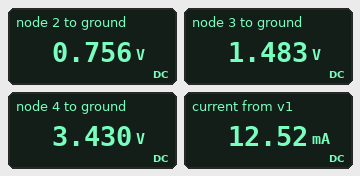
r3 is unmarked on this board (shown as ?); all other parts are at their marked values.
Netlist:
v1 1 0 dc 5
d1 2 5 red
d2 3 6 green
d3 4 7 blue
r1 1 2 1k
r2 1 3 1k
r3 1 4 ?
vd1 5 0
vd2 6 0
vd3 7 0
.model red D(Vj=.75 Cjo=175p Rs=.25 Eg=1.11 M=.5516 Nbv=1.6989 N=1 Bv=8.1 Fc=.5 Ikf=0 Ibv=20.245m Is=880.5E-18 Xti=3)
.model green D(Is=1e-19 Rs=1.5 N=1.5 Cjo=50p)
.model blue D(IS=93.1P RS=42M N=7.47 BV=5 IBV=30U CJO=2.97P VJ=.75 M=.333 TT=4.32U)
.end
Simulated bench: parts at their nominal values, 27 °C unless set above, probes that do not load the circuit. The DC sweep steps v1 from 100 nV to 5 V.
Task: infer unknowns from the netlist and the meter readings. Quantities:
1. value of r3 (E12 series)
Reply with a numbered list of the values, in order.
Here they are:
1. 330 Ω
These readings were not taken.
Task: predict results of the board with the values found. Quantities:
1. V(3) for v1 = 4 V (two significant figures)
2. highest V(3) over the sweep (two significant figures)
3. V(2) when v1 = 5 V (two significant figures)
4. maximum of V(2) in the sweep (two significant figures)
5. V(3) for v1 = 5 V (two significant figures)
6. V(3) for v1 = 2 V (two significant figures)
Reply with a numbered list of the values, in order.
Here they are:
1. 1.5 V
2. 1.5 V
3. 760 mV
4. 760 mV
5. 1.5 V
6. 1.4 V
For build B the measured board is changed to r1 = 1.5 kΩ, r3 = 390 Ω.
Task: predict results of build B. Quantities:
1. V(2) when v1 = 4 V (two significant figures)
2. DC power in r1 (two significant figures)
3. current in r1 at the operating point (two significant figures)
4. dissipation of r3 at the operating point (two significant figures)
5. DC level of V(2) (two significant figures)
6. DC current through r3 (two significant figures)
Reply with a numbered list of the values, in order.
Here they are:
1. 740 mV
2. 12 mW
3. 2.8 mA
4. 6.6 mW
5. 750 mV
6. 4.1 mA
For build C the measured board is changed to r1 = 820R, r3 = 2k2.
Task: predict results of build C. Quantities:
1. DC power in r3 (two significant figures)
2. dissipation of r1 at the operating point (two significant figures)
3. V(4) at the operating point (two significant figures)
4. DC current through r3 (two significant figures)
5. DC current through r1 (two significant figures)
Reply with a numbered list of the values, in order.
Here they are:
1. 1.6 mW
2. 22 mW
3. 3.1 V
4. 860 µA
5. 5.2 mA
